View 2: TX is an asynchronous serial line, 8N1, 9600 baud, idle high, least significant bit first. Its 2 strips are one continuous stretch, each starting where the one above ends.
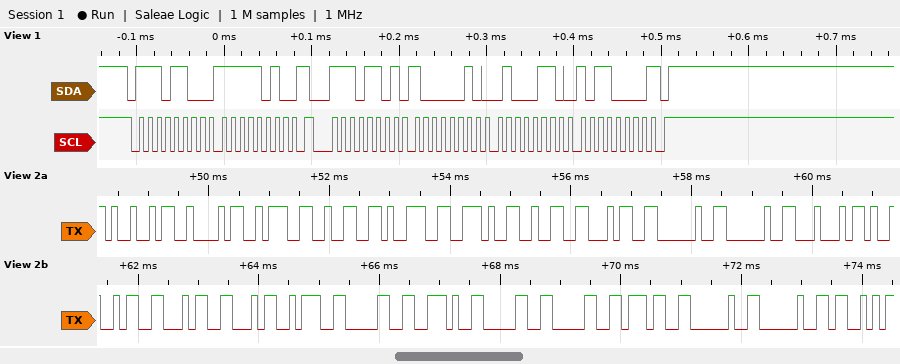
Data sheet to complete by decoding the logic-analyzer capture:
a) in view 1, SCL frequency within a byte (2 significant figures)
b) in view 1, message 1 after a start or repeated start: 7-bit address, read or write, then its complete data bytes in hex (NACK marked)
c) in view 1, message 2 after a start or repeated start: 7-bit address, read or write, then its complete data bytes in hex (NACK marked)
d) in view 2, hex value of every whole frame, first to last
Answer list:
100 kHz
0x76 write: FA
0x76 read: 82 46 B0 NACK
0x49 0x42 0x3A 0x32 0x39 0x2E 0x32 0x34 0x20 0x20 0x44 0x49 0x46 0x46 0x3A 0x30 0x2E 0x30 0x30 0x37 0x20 0x20 0x53
